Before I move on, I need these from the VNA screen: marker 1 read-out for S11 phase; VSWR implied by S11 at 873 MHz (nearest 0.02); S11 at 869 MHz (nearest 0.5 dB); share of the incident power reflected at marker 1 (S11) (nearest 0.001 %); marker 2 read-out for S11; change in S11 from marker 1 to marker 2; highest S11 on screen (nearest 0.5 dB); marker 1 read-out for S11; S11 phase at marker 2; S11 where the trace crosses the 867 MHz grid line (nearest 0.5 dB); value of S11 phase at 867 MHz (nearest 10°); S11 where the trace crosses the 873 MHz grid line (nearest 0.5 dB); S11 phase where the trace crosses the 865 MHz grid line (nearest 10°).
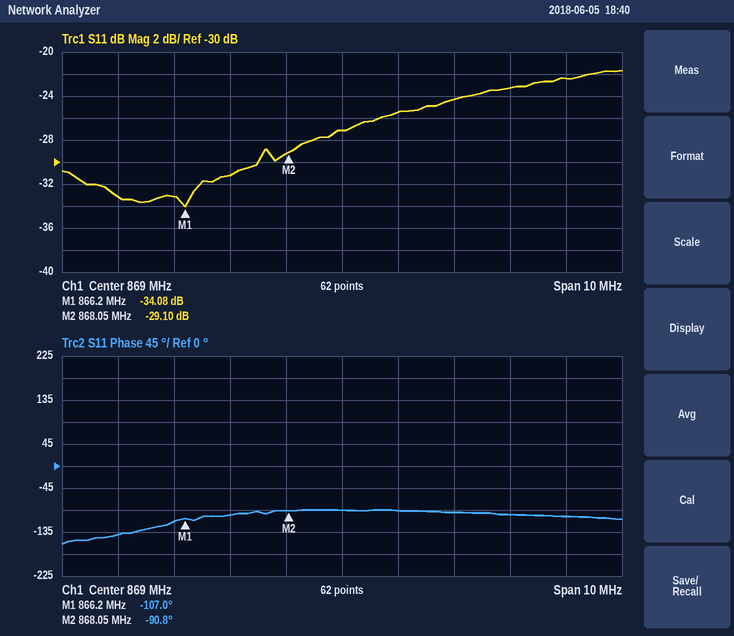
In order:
-107.0°
1.16
-27.0 dB
0.039 %
-29.10 dB
4.98 dB
-21.5 dB
-34.08 dB
-90.8°
-31.0 dB
-100°
-22.5 dB
-140°
